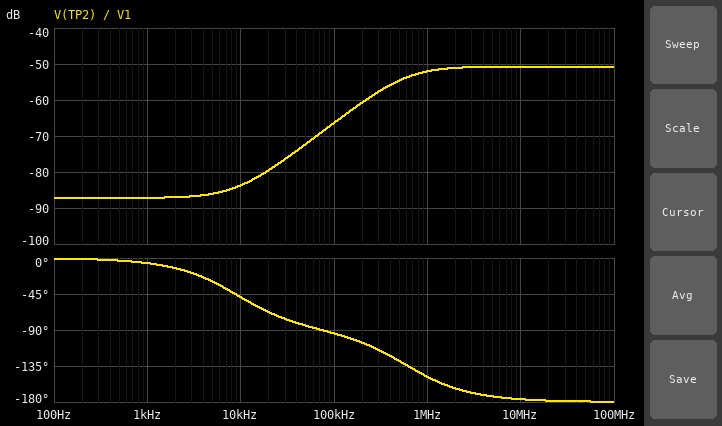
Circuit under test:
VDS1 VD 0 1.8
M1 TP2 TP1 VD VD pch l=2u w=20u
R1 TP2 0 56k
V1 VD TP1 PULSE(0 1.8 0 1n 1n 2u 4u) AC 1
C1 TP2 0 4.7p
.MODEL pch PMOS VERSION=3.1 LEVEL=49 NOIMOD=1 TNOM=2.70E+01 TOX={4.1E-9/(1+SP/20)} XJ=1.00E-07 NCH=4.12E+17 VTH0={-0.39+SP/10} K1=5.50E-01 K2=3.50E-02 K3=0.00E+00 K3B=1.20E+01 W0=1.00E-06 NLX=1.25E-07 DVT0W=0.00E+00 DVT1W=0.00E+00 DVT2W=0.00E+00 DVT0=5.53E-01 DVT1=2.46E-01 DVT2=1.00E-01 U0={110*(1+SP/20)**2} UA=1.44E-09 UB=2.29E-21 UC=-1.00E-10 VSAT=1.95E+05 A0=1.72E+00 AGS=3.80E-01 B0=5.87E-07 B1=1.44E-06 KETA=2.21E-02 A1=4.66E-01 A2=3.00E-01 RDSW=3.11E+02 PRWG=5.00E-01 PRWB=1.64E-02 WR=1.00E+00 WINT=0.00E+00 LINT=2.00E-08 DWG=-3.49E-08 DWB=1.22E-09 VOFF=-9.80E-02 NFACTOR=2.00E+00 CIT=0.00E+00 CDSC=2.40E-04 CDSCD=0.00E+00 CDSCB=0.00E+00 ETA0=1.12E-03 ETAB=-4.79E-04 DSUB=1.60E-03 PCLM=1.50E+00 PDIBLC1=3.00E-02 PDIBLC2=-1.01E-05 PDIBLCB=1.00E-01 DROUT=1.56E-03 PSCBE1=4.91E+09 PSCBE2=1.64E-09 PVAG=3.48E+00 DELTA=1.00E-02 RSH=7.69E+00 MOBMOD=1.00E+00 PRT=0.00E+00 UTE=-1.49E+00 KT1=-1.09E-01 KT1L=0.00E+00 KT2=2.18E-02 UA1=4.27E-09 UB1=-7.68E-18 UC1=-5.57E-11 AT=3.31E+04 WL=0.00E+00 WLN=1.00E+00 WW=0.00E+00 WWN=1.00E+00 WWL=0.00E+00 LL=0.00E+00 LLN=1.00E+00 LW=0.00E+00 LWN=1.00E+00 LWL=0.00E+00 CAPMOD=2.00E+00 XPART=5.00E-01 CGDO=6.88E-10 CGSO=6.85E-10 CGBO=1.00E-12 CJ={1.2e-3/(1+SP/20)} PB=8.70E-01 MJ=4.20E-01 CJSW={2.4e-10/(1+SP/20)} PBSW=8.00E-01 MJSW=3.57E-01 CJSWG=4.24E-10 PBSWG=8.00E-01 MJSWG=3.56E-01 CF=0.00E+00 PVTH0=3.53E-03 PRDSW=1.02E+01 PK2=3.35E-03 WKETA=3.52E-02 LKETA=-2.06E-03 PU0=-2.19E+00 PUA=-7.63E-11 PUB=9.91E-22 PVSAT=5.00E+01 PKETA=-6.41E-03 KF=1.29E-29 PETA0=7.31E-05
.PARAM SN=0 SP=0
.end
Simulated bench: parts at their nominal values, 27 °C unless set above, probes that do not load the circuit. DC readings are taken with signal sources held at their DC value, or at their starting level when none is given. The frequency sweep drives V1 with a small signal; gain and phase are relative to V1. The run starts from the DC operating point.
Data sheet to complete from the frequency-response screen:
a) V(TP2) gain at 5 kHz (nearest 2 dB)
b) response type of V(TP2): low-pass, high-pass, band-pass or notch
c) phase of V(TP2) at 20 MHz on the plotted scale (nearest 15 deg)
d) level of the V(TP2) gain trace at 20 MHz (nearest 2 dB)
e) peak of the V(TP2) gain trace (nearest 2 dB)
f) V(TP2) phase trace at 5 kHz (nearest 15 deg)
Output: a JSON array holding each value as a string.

["-86 dB", "high-pass", "-180 deg", "-50 dB", "-50 dB", "-30 deg"]
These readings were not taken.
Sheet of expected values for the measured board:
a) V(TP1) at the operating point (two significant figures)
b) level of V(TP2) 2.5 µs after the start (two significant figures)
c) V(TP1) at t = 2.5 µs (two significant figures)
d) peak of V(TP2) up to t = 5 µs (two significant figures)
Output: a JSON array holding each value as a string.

["1.8 V", "270 mV", "1.8 V", "1.8 V"]
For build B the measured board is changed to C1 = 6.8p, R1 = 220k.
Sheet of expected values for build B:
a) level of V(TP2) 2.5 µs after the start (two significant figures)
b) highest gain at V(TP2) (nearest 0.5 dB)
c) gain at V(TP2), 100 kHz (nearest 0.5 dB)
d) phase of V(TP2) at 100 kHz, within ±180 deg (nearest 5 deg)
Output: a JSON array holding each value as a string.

["1.3 V", "-54.0 dB", "-57.0 dB", "-130 deg"]
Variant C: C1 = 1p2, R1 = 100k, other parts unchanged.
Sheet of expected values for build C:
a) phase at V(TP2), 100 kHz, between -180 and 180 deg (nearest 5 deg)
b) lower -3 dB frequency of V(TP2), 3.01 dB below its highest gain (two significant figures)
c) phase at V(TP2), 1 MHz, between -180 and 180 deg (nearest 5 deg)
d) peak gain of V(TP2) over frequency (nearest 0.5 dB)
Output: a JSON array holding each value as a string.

["-90 deg", "1.3 MHz", "-125 deg", "-39.0 dB"]
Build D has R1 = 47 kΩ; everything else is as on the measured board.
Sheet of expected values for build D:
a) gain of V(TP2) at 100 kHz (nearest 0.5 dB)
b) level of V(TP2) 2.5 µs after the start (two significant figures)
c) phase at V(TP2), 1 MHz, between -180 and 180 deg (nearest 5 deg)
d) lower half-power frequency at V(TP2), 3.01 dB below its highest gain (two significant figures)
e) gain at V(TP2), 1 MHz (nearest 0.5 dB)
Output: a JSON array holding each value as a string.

["-68.0 dB", "190 mV", "-145 deg", "720 kHz", "-52.5 dB"]
